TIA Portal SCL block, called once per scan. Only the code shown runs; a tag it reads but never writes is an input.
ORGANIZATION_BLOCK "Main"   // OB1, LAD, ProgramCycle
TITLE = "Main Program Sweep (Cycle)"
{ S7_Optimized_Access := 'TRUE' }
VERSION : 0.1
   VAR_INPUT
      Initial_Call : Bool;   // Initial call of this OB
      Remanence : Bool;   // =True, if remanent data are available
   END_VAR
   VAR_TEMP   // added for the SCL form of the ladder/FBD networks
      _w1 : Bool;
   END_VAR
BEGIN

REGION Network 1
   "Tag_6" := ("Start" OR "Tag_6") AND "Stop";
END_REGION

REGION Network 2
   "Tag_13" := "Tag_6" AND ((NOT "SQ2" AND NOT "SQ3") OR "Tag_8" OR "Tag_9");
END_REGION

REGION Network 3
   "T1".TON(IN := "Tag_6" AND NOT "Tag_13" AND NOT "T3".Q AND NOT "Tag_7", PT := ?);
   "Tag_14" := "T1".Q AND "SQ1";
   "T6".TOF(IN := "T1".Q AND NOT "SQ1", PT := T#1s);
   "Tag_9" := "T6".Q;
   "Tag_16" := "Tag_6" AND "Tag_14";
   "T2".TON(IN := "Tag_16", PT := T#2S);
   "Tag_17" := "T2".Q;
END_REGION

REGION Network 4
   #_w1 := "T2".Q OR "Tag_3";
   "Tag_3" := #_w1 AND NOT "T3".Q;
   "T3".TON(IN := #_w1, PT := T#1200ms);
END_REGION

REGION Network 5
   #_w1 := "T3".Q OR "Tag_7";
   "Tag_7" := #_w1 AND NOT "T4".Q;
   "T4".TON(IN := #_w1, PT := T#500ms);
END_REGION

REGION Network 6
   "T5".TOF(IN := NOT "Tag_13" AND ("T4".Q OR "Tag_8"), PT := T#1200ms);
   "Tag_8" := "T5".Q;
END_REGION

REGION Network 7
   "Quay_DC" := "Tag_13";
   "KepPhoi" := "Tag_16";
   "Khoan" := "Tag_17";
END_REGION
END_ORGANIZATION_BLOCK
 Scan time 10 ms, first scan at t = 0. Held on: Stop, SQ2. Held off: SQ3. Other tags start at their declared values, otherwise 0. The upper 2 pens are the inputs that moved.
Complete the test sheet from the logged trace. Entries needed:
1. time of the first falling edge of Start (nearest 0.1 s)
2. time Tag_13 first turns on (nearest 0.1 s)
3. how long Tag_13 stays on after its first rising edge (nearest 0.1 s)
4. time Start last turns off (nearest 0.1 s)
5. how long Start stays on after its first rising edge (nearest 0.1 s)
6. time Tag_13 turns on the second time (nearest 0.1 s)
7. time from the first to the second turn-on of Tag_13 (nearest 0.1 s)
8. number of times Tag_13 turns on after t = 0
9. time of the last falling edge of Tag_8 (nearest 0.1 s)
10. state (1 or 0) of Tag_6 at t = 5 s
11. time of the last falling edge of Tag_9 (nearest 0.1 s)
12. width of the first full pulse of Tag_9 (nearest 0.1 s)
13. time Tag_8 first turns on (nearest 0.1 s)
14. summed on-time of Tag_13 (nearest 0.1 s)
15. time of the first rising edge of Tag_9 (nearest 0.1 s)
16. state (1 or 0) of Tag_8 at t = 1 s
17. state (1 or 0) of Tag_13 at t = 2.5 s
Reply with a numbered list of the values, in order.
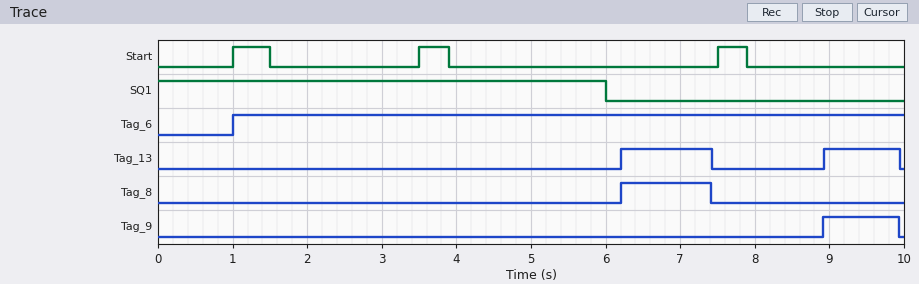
1. 1.5 s
2. 6.2 s
3. 1.2 s
4. 7.9 s
5. 0.5 s
6. 8.9 s
7. 2.7 s
8. 2
9. 7.4 s
10. 1
11. 9.9 s
12. 1.0 s
13. 6.2 s
14. 2.2 s
15. 8.9 s
16. 0
17. 0
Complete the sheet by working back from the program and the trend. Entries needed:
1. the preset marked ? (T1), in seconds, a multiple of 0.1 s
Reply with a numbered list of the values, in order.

1. 1.5 s
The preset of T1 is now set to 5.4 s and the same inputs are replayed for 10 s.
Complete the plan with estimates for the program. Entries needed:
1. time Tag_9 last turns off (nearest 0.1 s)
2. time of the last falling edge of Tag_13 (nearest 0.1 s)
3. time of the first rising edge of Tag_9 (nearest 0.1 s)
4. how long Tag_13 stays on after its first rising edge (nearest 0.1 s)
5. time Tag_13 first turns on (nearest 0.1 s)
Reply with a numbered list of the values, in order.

1. 7.4 s
2. 7.4 s
3. 6.4 s
4. 1.0 s
5. 6.4 s
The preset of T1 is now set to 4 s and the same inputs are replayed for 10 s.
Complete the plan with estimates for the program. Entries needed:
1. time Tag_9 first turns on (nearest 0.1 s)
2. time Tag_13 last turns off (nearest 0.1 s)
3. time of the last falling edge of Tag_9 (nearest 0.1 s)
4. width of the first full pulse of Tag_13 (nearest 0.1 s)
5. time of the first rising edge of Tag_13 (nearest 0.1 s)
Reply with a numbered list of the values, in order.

1. 6.0 s
2. 7.0 s
3. 7.0 s
4. 1.0 s
5. 6.0 s
